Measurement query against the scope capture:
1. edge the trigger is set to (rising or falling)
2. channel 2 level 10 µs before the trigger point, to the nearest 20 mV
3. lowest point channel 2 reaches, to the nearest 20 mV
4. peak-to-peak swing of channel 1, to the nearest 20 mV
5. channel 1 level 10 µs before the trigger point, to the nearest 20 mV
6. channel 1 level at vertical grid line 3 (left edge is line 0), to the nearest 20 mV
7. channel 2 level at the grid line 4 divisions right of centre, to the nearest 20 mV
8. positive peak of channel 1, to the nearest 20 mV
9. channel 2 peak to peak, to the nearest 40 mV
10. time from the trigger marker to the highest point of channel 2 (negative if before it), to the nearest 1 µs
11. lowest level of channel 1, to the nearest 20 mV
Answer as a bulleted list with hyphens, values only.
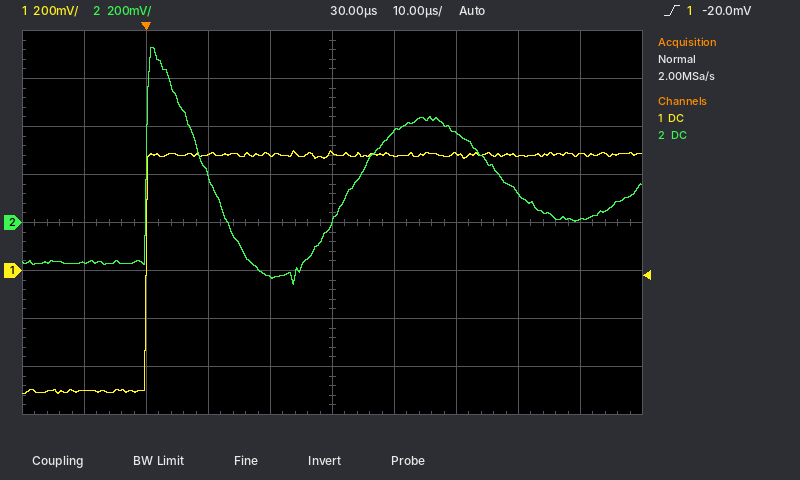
- rising
- -160 mV
- -260 mV
- 1.02 V
- -500 mV
- 480 mV
- 20 mV
- 500 mV
- 1.00 V
- +1 µs
- -520 mV
